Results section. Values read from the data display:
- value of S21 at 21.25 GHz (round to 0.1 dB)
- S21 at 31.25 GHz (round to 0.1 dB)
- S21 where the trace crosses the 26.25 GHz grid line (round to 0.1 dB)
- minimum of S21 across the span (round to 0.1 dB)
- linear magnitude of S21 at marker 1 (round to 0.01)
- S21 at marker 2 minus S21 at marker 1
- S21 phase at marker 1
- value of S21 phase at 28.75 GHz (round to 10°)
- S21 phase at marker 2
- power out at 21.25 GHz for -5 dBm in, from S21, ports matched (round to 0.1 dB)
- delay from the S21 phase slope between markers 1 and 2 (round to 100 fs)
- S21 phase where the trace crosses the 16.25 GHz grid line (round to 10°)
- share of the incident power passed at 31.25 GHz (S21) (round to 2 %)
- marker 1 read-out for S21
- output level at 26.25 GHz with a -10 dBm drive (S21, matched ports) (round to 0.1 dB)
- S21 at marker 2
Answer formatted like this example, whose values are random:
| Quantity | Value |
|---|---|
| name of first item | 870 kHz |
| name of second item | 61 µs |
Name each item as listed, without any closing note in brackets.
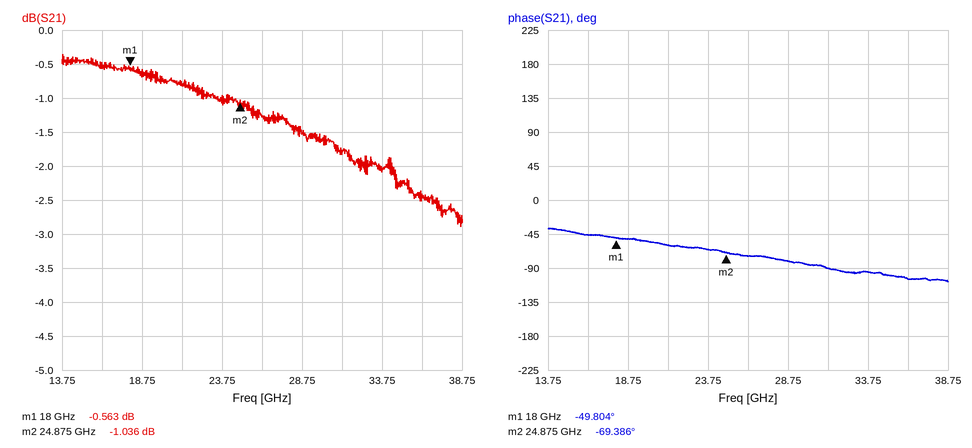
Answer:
| Quantity | Value |
|---|---|
| value of S21 at 21.25 GHz | -0.8 dB |
| S21 at 31.25 GHz | -1.8 dB |
| S21 where the trace crosses the 26.25 GHz grid line | -1.3 dB |
| minimum of S21 across the span | -2.9 dB |
| linear magnitude of S21 at marker 1 | 0.94 |
| S21 at marker 2 minus S21 at marker 1 | -0.473 dB |
| S21 phase at marker 1 | -49.804° |
| value of S21 phase at 28.75 GHz | -80° |
| S21 phase at marker 2 | -69.386° |
| power out at 21.25 GHz for -5 dBm in, from S21, ports matched | -5.8 dBm |
| delay from the S21 phase slope between markers 1 and 2 | 7.9 ps |
| S21 phase where the trace crosses the 16.25 GHz grid line | -50° |
| share of the incident power passed at 31.25 GHz (S21) | 66 % |
| marker 1 read-out for S21 | -0.563 dB |
| output level at 26.25 GHz with a -10 dBm drive (S21, matched ports) | -11.3 dBm |
| S21 at marker 2 | -1.036 dB |
